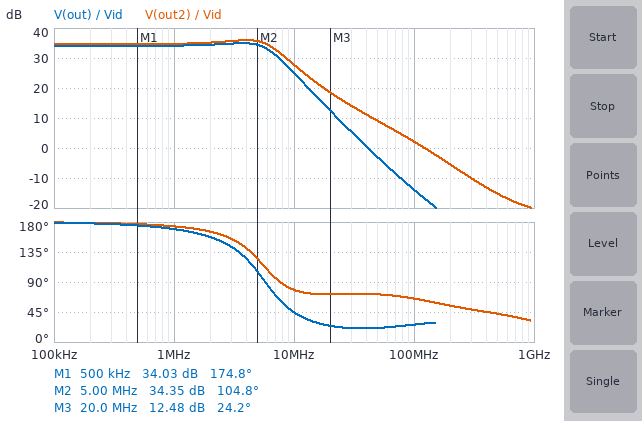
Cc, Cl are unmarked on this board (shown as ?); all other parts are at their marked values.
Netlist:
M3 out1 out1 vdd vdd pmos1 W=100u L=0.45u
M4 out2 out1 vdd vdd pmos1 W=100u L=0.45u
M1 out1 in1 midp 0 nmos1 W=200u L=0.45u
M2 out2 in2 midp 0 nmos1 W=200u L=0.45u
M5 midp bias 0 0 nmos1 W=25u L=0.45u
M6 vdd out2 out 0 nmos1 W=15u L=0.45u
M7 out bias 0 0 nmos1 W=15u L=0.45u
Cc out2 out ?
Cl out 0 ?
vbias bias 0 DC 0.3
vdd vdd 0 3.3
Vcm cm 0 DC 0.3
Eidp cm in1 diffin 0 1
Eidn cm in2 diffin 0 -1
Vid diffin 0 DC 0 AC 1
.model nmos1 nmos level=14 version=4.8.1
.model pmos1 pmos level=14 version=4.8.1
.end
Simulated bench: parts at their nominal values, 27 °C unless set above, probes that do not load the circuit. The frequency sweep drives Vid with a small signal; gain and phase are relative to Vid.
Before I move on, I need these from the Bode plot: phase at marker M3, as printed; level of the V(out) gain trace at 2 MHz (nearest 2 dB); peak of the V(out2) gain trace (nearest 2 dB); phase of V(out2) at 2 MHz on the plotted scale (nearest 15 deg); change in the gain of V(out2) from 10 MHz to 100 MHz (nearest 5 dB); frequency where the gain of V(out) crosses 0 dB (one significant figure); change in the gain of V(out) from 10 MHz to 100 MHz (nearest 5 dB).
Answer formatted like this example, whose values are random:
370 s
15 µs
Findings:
24.2 deg
34 dB
36 dB
165 deg
-25 dB
40 MHz
-40 dB
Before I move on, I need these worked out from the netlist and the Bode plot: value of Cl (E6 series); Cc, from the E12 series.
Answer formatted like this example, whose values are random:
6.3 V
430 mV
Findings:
22 pF
2.7 pF
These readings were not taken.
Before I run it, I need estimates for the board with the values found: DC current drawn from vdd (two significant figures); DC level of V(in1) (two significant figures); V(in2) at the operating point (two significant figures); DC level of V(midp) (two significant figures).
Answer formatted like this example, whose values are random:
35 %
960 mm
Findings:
190 µA
300 mV
300 mV
130 mV
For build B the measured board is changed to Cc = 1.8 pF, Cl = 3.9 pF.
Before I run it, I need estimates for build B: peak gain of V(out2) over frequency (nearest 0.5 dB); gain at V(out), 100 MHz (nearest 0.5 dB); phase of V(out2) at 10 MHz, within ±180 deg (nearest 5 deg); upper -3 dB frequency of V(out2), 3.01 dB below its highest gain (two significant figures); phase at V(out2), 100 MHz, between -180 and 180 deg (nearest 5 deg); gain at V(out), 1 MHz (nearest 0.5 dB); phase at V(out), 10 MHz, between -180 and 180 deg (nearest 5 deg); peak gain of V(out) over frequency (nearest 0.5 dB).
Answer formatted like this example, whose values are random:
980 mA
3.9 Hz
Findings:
34.5 dB
1.5 dB
125 deg
12 MHz
55 deg
34.0 dB
115 deg
34.0 dB
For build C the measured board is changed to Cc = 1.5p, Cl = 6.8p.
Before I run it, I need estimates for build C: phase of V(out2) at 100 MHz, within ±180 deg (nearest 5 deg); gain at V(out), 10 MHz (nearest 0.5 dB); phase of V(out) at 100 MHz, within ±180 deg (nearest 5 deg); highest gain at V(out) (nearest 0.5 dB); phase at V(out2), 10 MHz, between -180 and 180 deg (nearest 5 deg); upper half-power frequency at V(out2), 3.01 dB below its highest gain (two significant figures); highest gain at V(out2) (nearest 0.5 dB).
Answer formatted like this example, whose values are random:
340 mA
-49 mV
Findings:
60 deg
32.0 dB
20 deg
34.0 dB
120 deg
12 MHz
34.5 dB
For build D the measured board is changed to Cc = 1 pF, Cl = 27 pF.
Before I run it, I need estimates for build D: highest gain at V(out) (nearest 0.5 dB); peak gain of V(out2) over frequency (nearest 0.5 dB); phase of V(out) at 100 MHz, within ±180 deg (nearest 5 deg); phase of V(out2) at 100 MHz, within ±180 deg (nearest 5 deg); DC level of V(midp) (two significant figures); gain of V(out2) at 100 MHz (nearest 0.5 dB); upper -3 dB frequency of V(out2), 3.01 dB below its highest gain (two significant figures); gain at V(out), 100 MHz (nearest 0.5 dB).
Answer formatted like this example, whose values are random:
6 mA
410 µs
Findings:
34.0 dB
35.0 dB
5 deg
70 deg
130 mV
7.5 dB
9.0 MHz
-12.0 dB
